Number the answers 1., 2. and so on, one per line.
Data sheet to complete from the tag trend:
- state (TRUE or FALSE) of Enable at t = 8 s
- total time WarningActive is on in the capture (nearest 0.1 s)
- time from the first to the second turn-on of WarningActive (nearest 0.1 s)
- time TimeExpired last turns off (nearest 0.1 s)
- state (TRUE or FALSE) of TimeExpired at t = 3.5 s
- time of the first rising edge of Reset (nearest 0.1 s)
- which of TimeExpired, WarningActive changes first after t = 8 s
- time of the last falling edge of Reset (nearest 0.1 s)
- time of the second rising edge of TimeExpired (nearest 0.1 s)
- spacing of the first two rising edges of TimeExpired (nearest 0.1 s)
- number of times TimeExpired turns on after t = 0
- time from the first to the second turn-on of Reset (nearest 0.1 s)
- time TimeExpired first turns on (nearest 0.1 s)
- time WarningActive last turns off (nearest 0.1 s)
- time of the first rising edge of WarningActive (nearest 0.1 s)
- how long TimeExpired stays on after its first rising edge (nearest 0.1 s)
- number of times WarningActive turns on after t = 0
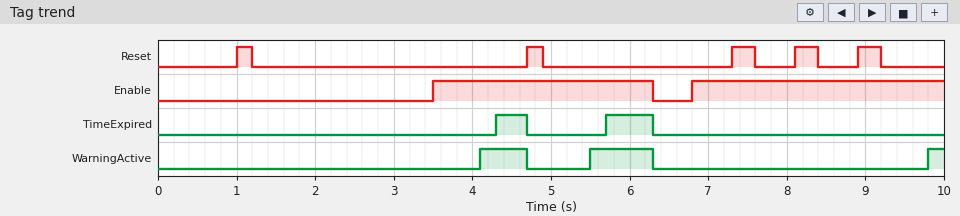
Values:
1. TRUE
2. 1.6 s
3. 1.4 s
4. 6.3 s
5. FALSE
6. 1.0 s
7. WarningActive
8. 9.2 s
9. 5.7 s
10. 1.4 s
11. 2
12. 3.7 s
13. 4.3 s
14. 6.3 s
15. 4.1 s
16. 0.4 s
17. 3
